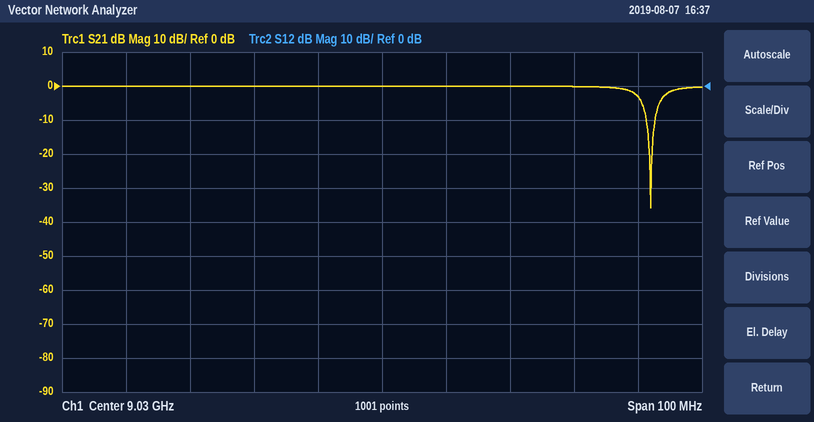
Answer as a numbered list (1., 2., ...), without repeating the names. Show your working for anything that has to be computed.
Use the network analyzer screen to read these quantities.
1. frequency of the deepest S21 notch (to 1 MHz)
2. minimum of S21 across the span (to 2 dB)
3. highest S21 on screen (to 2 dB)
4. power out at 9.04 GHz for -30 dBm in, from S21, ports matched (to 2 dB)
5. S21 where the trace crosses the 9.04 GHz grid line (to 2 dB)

1. 9.072 GHz
2. -36 dB
3. 0 dB
4. -30 dBm + (0 dB) = -30 dBm
5. 0 dB
